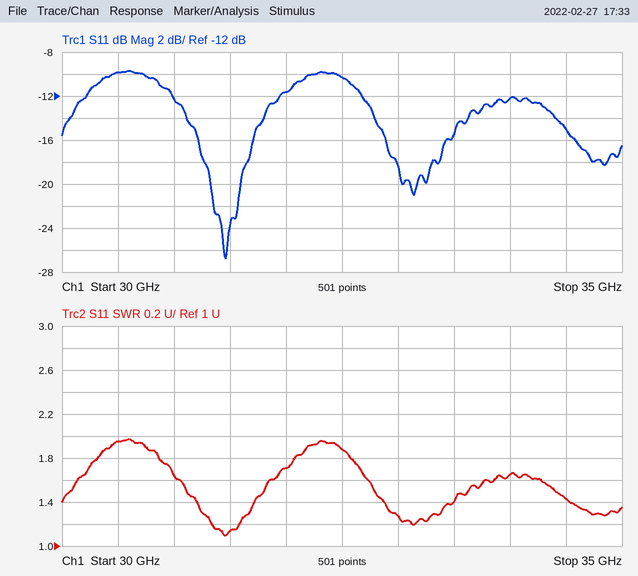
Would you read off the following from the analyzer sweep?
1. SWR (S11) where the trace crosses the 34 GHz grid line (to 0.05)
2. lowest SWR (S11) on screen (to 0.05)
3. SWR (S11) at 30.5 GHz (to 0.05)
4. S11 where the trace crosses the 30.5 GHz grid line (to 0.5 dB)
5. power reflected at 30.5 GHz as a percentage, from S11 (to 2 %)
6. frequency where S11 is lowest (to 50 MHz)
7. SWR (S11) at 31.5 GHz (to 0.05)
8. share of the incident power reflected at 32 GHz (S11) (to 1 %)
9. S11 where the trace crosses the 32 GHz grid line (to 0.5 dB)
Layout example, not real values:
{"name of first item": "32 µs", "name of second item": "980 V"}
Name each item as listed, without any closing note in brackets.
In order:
{"SWR (S11) where the trace crosses the 34 GHz grid line": "1.65", "lowest SWR (S11) on screen": "1.10", "SWR (S11) at 30.5 GHz": "1.95", "S11 where the trace crosses the 30.5 GHz grid line": "-10.0 dB", "power reflected at 30.5 GHz as a percentage, from S11": "10 %", "frequency where S11 is lowest": "31.45 GHz", "SWR (S11) at 31.5 GHz": "1.15", "share of the incident power reflected at 32 GHz (S11)": "7 %", "S11 where the trace crosses the 32 GHz grid line": "-11.5 dB"}
